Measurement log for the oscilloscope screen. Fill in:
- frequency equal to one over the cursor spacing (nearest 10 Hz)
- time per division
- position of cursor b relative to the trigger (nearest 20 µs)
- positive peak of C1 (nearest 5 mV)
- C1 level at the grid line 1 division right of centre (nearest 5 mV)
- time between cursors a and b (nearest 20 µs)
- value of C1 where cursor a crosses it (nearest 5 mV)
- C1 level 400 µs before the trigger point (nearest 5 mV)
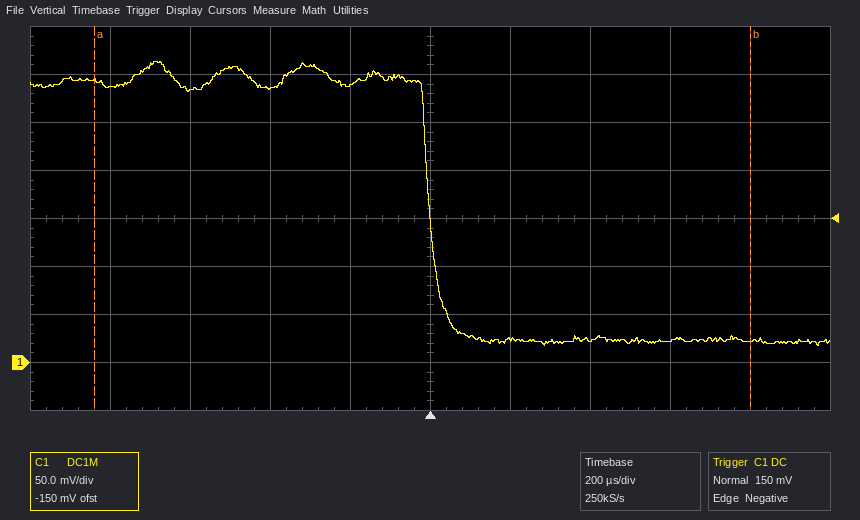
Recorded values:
610 Hz
200 µs
+800 µs
315 mV
25 mV
1.64 ms
295 mV
285 mV
